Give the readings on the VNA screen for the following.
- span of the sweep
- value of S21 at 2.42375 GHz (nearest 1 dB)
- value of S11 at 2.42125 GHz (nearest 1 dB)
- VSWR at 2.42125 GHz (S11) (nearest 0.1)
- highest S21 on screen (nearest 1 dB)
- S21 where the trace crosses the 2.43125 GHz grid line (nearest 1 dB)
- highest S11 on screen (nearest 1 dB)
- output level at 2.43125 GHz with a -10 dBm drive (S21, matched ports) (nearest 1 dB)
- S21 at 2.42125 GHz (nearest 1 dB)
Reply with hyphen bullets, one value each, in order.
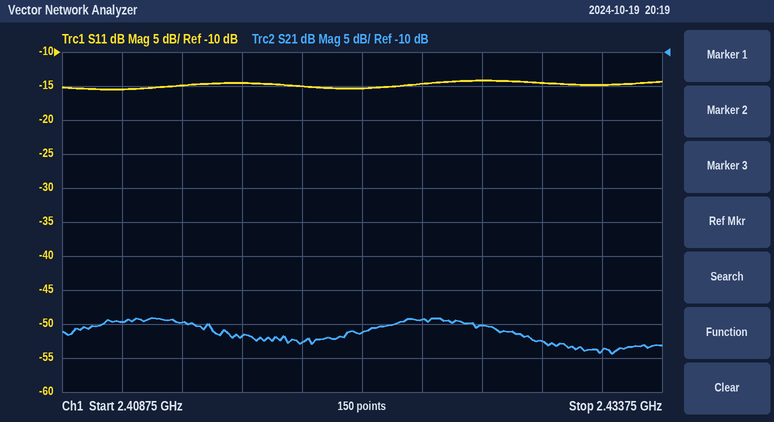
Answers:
- 25 MHz
- -49 dB
- -15 dB
- 1.4
- -49 dB
- -54 dB
- -14 dB
- -64 dBm
- -51 dB
